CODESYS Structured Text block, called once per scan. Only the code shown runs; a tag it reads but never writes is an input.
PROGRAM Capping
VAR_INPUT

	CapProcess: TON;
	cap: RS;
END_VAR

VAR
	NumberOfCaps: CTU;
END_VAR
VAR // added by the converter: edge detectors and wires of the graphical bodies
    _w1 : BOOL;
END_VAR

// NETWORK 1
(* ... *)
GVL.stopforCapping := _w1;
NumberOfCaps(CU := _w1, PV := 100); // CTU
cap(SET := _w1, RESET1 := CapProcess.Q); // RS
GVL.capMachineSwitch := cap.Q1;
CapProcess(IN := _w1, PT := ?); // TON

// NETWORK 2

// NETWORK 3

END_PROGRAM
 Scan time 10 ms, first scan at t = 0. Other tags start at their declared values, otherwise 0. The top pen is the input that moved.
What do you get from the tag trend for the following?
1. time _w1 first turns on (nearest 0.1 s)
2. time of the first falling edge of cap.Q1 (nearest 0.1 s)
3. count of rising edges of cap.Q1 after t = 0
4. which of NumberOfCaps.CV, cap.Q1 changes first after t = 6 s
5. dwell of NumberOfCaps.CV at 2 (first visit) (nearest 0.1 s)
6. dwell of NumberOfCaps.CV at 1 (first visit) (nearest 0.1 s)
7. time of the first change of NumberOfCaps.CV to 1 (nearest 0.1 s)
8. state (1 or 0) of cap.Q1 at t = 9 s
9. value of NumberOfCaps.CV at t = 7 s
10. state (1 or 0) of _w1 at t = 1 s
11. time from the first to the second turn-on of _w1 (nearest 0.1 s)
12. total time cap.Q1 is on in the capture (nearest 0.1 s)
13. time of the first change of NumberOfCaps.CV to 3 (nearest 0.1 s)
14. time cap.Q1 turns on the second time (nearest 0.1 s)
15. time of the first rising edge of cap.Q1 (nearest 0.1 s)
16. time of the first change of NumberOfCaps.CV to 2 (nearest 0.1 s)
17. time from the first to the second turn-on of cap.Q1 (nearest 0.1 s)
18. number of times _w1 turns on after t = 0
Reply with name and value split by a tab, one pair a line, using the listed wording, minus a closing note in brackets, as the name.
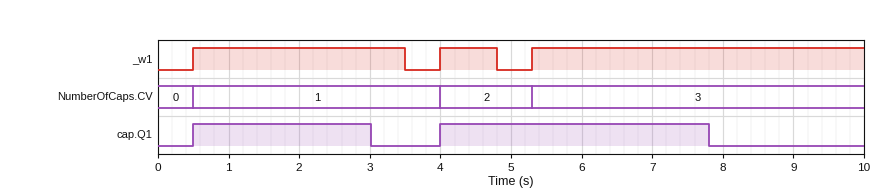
time _w1 first turns on	0.5 s
time of the first falling edge of cap.Q1	3.0 s
count of rising edges of cap.Q1 after t = 0	2
which of NumberOfCaps.CV, cap.Q1 changes first after t = 6 s	cap.Q1
dwell of NumberOfCaps.CV at 2 (first visit)	1.3 s
dwell of NumberOfCaps.CV at 1 (first visit)	3.5 s
time of the first change of NumberOfCaps.CV to 1	0.5 s
state (1 or 0) of cap.Q1 at t = 9 s	0
value of NumberOfCaps.CV at t = 7 s	3
state (1 or 0) of _w1 at t = 1 s	1
time from the first to the second turn-on of _w1	3.5 s
total time cap.Q1 is on in the capture	6.3 s
time of the first change of NumberOfCaps.CV to 3	5.3 s
time cap.Q1 turns on the second time	4.0 s
time of the first rising edge of cap.Q1	0.5 s
time of the first change of NumberOfCaps.CV to 2	4.0 s
time from the first to the second turn-on of cap.Q1	3.5 s
number of times _w1 turns on after t = 0	3
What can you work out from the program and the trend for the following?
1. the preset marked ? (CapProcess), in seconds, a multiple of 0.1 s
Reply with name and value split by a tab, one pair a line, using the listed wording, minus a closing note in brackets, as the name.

the preset marked ? (CapProcess), in seconds, a multiple of 0.1 s	2.5 s
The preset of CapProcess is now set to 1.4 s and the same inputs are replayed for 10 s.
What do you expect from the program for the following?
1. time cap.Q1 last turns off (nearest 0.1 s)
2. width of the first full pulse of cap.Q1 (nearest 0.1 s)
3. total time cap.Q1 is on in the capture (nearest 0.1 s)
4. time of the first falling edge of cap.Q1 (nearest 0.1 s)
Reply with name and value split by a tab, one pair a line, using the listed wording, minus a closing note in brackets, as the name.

time cap.Q1 last turns off	6.7 s
width of the first full pulse of cap.Q1	1.4 s
total time cap.Q1 is on in the capture	4.1 s
time of the first falling edge of cap.Q1	1.9 s
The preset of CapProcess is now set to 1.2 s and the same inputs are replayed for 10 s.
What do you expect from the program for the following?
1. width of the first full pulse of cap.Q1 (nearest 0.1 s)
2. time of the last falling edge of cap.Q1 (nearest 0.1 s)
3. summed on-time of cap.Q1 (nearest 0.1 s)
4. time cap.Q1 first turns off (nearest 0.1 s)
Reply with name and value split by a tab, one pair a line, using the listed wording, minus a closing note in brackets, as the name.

width of the first full pulse of cap.Q1	1.2 s
time of the last falling edge of cap.Q1	6.5 s
summed on-time of cap.Q1	3.7 s
time cap.Q1 first turns off	1.7 s
